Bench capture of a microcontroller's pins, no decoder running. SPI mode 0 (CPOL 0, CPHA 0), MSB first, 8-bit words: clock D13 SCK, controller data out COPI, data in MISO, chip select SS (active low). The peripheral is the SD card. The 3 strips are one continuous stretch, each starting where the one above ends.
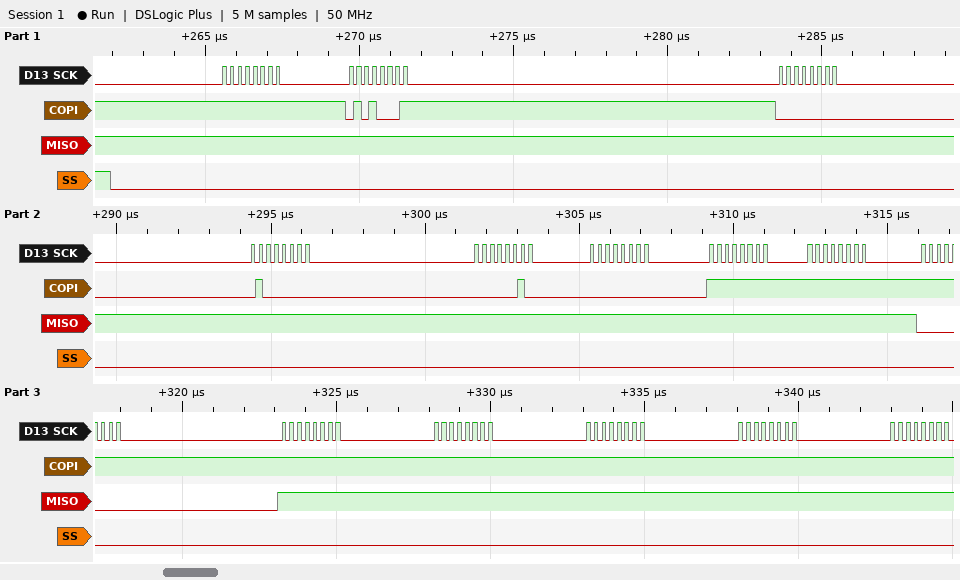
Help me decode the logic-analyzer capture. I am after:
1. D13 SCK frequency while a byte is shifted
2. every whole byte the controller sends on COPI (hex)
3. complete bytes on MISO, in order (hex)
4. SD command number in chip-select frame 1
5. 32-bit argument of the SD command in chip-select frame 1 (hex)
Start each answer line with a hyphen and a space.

- 4 MHz
- FF 51 00 40 02 00 FF FF FF FF FF FF FF FF
- FF FF FF FF FF FF FF FF 00 FF FF FF FF FF
- CMD17
- 0x00400200
